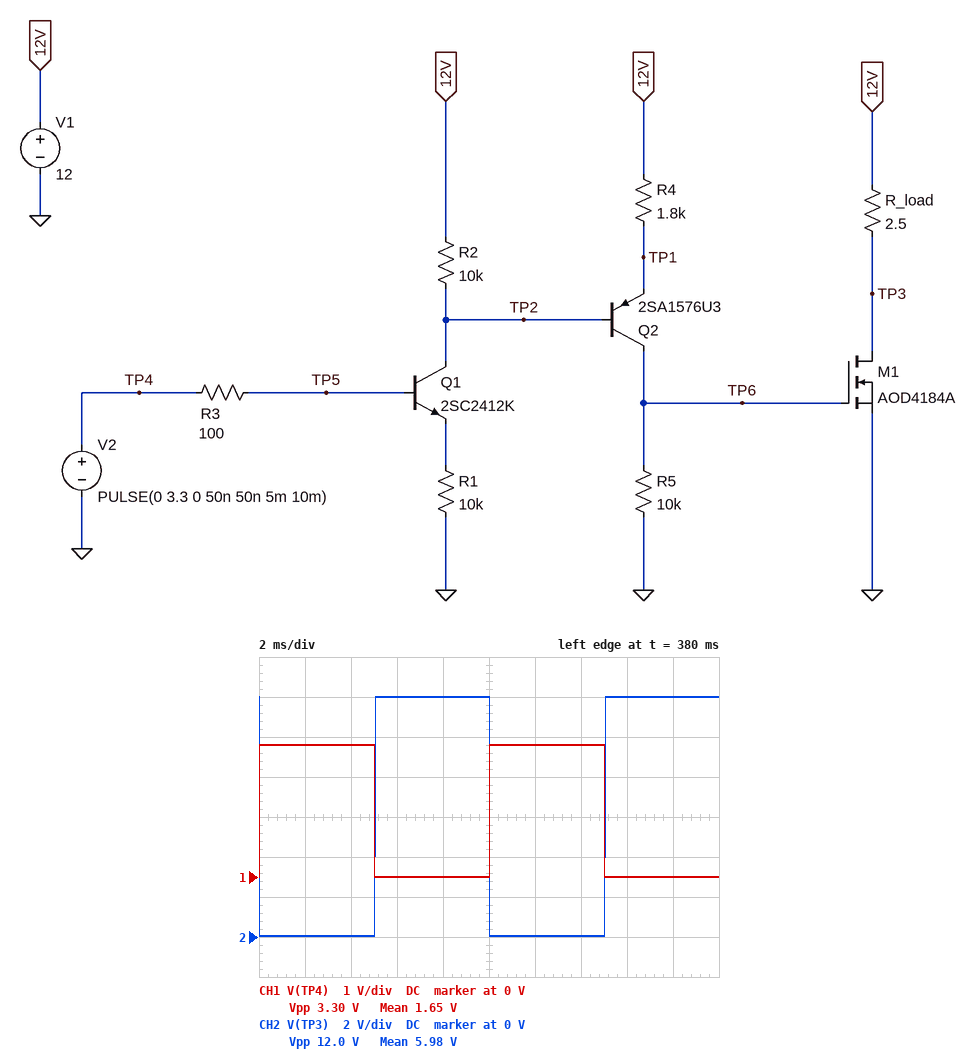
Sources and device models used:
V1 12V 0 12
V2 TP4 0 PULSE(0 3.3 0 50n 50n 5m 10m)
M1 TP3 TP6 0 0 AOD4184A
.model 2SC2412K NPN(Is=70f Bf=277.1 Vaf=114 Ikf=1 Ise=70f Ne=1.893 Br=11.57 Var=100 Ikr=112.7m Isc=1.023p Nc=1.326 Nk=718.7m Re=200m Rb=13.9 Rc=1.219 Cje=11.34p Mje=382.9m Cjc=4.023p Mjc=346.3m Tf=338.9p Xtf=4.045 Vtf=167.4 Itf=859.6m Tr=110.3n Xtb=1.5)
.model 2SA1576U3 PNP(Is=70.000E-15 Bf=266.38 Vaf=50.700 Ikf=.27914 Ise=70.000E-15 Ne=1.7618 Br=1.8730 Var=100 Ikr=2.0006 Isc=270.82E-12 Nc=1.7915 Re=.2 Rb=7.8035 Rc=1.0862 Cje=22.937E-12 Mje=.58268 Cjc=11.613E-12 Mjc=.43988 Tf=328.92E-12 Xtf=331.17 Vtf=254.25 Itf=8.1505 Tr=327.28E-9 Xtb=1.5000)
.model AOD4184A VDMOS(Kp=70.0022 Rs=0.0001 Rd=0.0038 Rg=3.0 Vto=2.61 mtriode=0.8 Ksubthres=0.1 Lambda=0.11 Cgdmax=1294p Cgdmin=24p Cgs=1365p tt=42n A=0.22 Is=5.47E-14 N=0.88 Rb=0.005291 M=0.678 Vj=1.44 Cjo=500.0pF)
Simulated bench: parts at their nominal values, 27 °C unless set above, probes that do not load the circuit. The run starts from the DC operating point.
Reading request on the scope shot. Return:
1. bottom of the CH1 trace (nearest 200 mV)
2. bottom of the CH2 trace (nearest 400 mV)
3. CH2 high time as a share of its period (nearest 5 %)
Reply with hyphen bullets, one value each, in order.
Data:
- 0 V
- 0 V
- 50 %
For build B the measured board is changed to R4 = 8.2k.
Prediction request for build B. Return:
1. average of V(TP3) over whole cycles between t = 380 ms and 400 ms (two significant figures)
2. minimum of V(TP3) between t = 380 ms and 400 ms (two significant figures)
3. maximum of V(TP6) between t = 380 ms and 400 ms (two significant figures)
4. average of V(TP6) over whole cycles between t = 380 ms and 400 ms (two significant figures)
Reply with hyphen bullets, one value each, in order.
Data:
- 12 V
- 11 V
- 2.6 V
- 1.3 V
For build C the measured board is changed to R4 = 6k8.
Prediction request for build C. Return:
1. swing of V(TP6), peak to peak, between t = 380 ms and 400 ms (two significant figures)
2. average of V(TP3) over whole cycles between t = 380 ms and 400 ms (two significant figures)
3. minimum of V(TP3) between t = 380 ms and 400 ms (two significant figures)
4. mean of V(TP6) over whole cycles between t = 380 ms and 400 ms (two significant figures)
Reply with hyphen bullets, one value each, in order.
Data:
- 3.1 V
- 6.2 V
- 200 mV
- 1.6 V
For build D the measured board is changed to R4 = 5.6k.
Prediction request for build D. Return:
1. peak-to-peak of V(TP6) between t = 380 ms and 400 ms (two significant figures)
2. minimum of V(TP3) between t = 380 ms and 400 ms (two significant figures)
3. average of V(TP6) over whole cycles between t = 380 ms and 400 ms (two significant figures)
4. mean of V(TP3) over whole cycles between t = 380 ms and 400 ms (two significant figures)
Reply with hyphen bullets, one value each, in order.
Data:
- 3.8 V
- 92 mV
- 1.9 V
- 6.1 V
